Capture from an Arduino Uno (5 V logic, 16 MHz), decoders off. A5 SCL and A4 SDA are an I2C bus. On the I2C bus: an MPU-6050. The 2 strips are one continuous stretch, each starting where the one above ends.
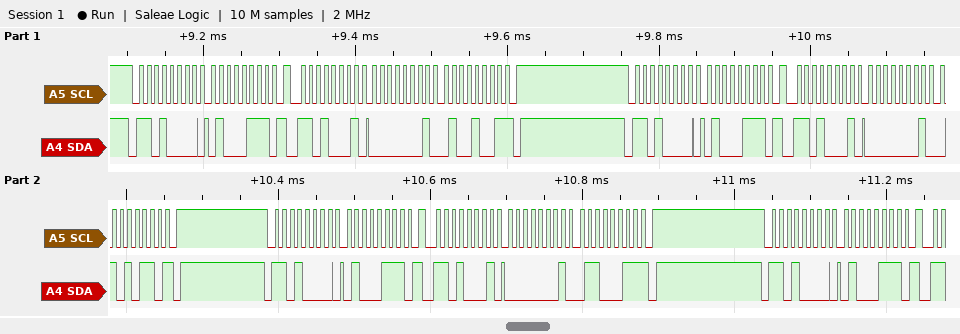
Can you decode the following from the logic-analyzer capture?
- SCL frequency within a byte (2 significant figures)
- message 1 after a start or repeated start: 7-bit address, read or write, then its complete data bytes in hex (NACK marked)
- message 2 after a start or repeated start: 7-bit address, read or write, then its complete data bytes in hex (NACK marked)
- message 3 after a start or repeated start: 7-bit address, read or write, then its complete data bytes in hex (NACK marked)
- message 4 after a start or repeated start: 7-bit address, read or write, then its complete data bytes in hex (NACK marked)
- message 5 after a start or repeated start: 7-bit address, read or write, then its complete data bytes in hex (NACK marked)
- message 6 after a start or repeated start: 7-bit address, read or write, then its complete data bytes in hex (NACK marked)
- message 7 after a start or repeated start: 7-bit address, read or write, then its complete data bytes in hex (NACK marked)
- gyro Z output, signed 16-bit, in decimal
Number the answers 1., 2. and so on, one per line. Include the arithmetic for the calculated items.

1. 100 kHz
2. 0x68 write: 47
3. 0x68 read: 01 49 NACK
4. 0x68 write: 47
5. 0x68 read: 01 56 NACK
6. 0x68 write: 47
7. 0x68 read: 01 63 NACK
8. 0x68 write: 47
9. 0x0149 = 329
